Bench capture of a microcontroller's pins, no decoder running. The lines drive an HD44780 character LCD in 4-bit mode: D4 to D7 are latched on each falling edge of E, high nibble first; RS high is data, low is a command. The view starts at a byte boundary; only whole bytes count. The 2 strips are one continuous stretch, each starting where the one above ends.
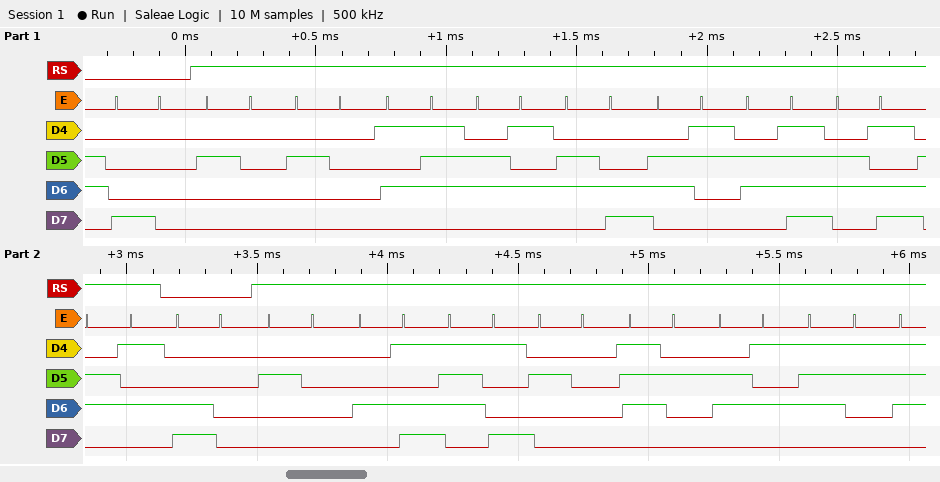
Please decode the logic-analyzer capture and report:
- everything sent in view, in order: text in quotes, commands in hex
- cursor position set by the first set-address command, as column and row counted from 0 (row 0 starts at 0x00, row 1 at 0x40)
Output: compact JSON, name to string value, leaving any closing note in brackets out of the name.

{"everything sent in view, in order: text in quotes, commands in hex": "0x80 \"  Welcome\" 0xC0 \" My res\"", "cursor position set by the first set-address command, as column and row counted from 0": "column 0, row 0"}
